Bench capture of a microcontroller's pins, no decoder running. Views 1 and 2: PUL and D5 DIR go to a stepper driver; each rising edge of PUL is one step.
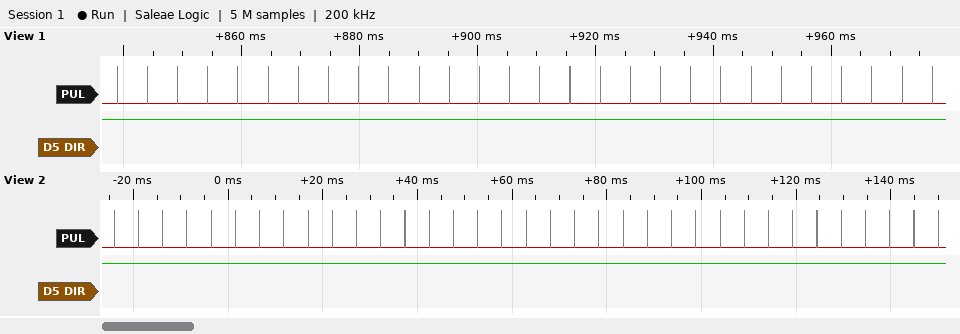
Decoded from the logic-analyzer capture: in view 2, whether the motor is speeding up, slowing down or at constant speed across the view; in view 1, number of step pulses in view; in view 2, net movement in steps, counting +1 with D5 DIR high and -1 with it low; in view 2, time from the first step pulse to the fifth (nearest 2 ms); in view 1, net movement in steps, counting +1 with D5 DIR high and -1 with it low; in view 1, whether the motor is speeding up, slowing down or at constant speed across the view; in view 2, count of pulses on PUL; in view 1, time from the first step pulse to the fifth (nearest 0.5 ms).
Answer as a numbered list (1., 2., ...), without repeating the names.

1. constant speed
2. 28
3. +35
4. 20 ms
5. +28
6. constant speed
7. 35
8. 20.5 ms
